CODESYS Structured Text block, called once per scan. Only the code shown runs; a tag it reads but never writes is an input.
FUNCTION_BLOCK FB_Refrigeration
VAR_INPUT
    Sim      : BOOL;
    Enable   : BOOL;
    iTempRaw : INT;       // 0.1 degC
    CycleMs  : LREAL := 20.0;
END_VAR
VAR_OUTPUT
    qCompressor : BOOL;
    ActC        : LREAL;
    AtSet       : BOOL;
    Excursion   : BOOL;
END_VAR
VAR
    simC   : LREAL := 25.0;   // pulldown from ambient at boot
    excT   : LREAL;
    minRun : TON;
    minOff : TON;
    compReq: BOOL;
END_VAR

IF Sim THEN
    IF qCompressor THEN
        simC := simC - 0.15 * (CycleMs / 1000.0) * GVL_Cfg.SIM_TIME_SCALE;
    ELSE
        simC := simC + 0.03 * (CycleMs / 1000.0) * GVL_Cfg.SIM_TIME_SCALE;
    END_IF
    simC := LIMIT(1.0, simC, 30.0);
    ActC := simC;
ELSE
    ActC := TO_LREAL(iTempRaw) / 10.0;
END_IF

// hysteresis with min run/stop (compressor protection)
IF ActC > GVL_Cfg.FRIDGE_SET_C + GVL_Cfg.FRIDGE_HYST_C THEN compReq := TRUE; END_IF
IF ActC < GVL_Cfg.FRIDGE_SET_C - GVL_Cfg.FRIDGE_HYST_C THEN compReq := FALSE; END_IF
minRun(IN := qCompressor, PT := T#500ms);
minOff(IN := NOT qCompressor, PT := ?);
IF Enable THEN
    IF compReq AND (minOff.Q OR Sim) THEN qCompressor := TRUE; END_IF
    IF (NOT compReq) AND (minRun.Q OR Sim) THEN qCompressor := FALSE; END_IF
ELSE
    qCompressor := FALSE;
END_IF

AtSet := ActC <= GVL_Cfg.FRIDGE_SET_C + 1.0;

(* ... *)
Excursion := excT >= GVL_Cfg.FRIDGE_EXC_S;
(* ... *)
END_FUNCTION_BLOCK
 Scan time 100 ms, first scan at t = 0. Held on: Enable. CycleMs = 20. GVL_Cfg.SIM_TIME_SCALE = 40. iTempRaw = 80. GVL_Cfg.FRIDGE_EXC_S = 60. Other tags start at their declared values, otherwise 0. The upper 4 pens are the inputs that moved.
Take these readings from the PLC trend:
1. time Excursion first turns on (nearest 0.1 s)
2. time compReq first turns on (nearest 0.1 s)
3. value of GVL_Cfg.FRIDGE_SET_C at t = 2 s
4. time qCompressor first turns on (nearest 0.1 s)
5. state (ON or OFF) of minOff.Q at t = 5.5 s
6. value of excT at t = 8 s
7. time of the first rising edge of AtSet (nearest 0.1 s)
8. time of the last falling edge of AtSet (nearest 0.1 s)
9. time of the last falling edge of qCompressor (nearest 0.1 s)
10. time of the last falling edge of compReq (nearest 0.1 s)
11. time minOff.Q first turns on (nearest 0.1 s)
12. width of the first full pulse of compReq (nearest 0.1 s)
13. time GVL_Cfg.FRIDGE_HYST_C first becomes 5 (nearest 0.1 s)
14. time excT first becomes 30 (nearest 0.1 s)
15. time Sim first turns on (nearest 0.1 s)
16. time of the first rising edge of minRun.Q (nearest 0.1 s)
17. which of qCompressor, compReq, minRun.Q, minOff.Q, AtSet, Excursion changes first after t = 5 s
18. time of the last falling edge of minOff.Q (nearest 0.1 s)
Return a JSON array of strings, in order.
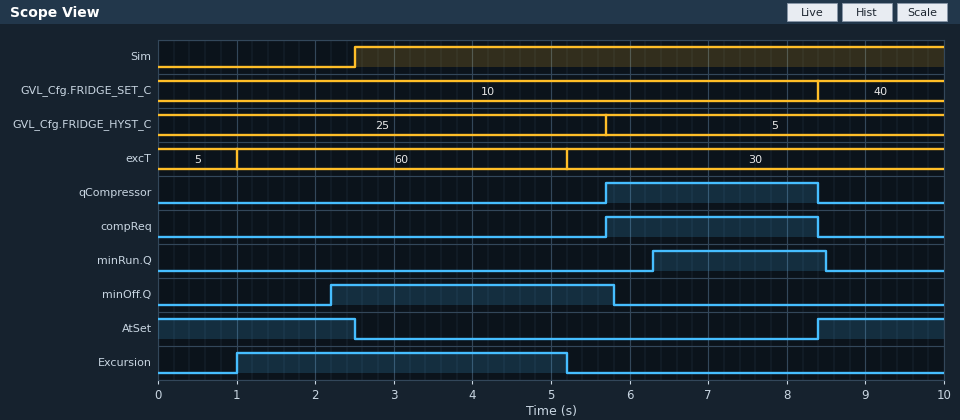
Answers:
["1.0 s", "5.7 s", "10", "5.7 s", "ON", "30", "8.4 s", "2.5 s", "8.4 s", "8.4 s", "2.2 s", "2.7 s", "5.7 s", "5.2 s", "2.5 s", "6.3 s", "Excursion", "5.8 s"]
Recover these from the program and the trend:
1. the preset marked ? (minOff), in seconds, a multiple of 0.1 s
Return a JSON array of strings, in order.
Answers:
["2.2 s"]
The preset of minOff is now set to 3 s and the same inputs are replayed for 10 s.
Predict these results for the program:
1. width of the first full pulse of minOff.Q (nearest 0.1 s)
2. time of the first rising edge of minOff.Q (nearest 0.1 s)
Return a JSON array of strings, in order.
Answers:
["2.8 s", "3.0 s"]
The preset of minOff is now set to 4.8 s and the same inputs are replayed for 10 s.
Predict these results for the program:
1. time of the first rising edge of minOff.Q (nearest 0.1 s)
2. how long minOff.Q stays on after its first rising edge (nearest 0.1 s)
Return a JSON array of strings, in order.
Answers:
["4.8 s", "1.0 s"]
